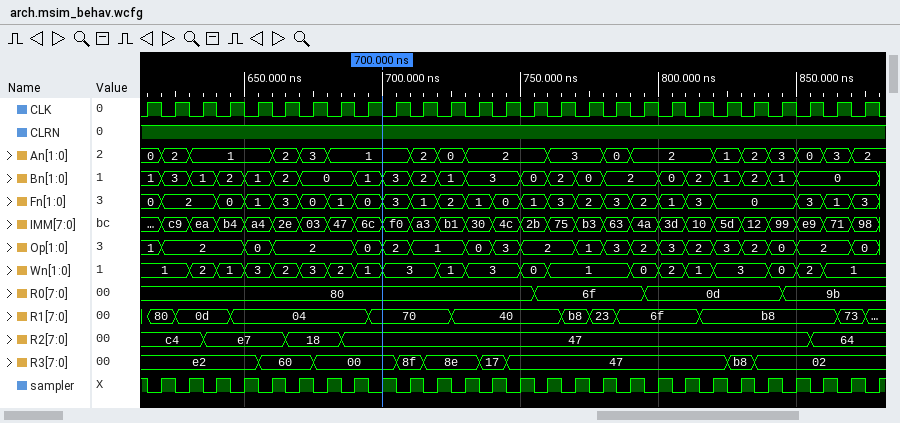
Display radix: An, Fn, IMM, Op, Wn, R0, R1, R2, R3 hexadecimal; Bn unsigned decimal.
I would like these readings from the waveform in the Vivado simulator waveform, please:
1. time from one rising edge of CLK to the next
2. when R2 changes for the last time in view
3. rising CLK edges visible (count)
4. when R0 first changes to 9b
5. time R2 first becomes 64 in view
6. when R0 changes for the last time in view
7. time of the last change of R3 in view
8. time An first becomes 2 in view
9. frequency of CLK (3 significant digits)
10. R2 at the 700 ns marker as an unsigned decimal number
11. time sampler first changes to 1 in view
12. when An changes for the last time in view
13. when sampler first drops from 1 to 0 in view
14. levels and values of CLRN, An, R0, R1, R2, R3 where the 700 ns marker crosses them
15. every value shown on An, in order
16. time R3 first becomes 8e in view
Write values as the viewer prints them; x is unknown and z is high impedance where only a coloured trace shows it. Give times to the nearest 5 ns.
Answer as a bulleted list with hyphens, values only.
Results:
- 10 ns
- 855 ns
- 27
- 845 ns
- 855 ns
- 845 ns
- 835 ns
- 620 ns
- 100 MHz
- 71
- 620 ns
- 870 ns
- 615 ns
- CLRN=1, An=1, R0=80, R1=70, R2=47, R3=00
- 0, 2, 1, 2, 3, 1, 2, 0, 2, 3, 0, 2, 1, 2, 3, 0, 3, 2
- 715 ns
